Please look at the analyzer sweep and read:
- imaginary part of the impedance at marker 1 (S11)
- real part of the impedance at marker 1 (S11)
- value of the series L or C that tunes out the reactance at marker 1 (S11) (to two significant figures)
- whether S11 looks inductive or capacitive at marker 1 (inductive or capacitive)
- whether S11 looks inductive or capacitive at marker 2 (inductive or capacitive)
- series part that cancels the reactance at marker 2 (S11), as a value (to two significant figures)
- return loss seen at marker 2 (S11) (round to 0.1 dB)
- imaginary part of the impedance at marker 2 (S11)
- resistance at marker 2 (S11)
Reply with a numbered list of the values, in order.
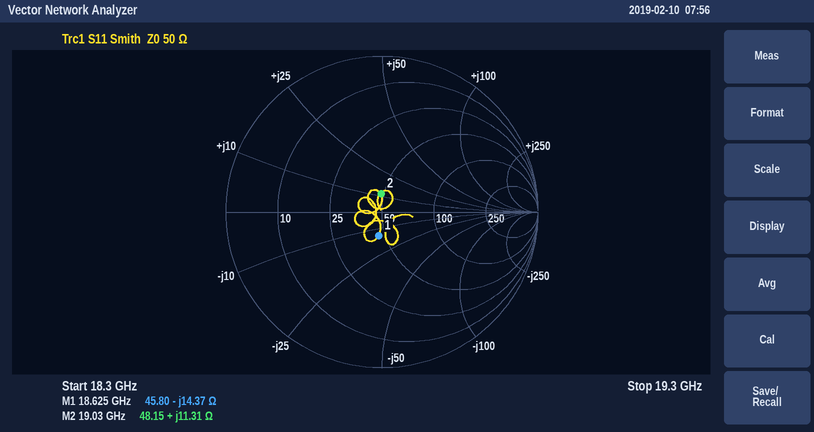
1. -14.37 Ω
2. 45.80 Ω
3. 120 pH
4. capacitive
5. inductive
6. 740 fF
7. 18.7 dB
8. +11.31 Ω
9. 48.15 Ω
